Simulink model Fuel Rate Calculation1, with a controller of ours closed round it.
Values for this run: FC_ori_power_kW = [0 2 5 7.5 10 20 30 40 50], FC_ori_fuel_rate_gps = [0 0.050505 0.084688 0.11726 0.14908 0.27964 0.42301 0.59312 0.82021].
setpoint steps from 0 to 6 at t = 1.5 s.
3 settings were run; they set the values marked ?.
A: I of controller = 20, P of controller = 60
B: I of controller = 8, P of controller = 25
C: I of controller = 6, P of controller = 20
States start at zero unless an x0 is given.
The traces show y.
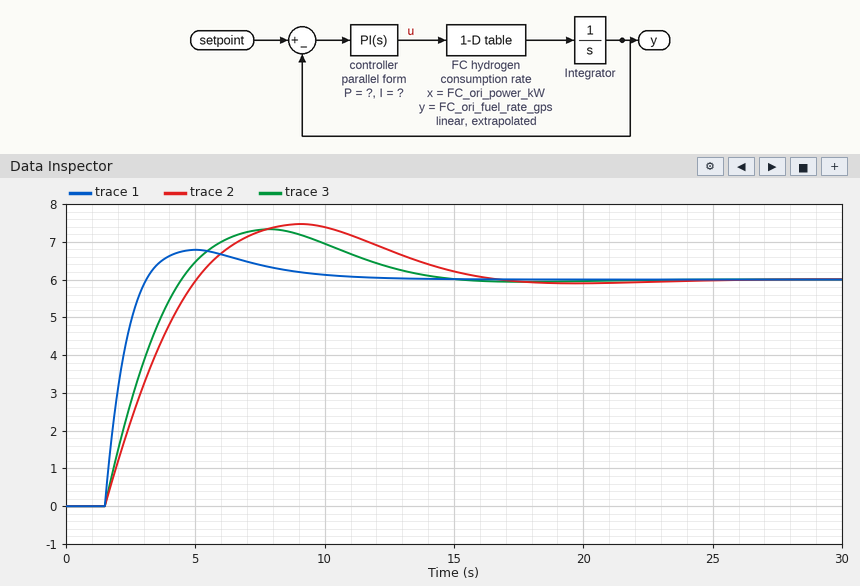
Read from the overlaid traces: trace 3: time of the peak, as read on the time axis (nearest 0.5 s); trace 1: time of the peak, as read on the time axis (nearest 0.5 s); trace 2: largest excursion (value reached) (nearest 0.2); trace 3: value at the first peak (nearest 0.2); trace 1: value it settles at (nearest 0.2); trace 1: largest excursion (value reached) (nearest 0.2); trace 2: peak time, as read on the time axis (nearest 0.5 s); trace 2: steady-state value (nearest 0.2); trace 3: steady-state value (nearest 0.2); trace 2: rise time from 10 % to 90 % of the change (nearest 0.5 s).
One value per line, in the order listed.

8.0 s
5.0 s
7.4
7.4
6.0
6.8
9.0 s
6.0
6.0
2.5 s
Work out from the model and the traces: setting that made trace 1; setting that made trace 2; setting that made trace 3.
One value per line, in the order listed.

A
C
B
